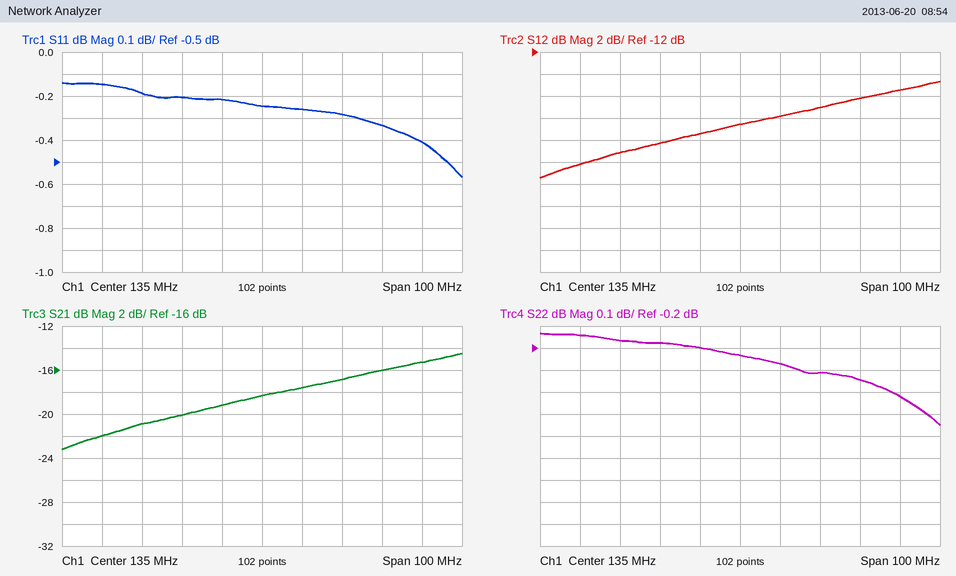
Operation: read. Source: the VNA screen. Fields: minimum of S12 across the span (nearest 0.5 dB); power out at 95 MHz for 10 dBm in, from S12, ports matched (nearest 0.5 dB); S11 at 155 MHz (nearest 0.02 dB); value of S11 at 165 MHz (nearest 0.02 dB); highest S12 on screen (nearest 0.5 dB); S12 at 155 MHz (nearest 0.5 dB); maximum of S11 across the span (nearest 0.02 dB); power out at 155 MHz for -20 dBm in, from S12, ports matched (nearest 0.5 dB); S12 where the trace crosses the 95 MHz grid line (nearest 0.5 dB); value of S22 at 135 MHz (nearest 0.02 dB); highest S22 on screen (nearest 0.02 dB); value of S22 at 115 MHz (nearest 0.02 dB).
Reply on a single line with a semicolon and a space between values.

-23.5 dB; -12.0 dBm; -0.28 dB; -0.34 dB; -14.5 dB; -17.0 dB; -0.14 dB; -37.0 dBm; -22.0 dB; -0.24 dB; -0.14 dB; -0.18 dB
